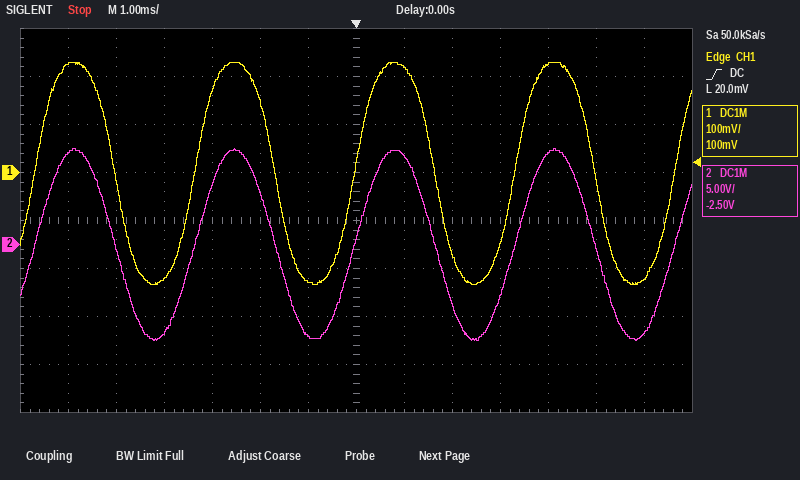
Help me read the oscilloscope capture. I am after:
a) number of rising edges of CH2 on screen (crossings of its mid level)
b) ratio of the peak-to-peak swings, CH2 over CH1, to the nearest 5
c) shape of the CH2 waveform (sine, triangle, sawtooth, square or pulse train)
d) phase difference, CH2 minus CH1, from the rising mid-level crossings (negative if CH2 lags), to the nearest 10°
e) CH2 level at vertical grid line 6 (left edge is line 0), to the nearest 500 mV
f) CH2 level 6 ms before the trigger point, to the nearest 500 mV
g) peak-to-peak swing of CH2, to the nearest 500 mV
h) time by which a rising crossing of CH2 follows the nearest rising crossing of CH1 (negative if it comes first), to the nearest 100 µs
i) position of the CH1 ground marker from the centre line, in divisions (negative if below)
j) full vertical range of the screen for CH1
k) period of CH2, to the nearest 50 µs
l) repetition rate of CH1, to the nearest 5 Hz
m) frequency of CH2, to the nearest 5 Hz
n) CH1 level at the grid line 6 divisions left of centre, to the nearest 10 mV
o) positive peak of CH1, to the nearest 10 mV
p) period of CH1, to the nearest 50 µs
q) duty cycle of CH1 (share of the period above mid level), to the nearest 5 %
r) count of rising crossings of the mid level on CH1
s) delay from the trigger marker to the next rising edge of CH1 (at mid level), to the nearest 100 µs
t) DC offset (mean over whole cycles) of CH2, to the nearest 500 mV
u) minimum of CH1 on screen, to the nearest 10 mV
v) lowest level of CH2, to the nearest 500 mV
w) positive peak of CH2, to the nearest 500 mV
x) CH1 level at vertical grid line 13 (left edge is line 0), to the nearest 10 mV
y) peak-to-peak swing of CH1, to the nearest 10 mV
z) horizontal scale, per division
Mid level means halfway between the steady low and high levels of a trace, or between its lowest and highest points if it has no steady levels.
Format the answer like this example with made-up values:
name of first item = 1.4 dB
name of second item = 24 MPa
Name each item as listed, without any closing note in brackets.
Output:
number of rising edges of CH2 on screen = 5
ratio of the peak-to-peak swings, CH2 over CH1, to the nearest 5 = 45
shape of the CH2 waveform = sine
phase difference, CH2 minus CH1, from the rising mid-level crossings (negative if CH2 lags), to the nearest 10° = 0°
CH2 level at vertical grid line 6 (left edge is line 0), to the nearest 500 mV = -9.5 V
CH2 level 6 ms before the trigger point, to the nearest 500 mV = 9.5 V
peak-to-peak swing of CH2, to the nearest 500 mV = 20.0 V
time by which a rising crossing of CH2 follows the nearest rising crossing of CH1 (negative if it comes first), to the nearest 100 µs = 0.0 ms
position of the CH1 ground marker from the centre line, in divisions = +1.0 div
full vertical range of the screen for CH1 = 800 mV
period of CH2, to the nearest 50 µs = 3.35 ms
repetition rate of CH1, to the nearest 5 Hz = 300 Hz
frequency of CH2, to the nearest 5 Hz = 300 Hz
CH1 level at the grid line 6 divisions left of centre, to the nearest 10 mV = 230 mV
positive peak of CH1, to the nearest 10 mV = 230 mV
period of CH1, to the nearest 50 µs = 3.35 ms
duty cycle of CH1 (share of the period above mid level), to the nearest 5 % = 50 %
count of rising crossings of the mid level on CH1 = 5
delay from the trigger marker to the next rising edge of CH1 (at mid level), to the nearest 100 µs = 3.3 ms
DC offset (mean over whole cycles) of CH2, to the nearest 500 mV = 0.0 V
minimum of CH1 on screen, to the nearest 10 mV = -230 mV
lowest level of CH2, to the nearest 500 mV = -10.0 V
positive peak of CH2, to the nearest 500 mV = 10.0 V
CH1 level at vertical grid line 13 (left edge is line 0), to the nearest 10 mV = -220 mV
peak-to-peak swing of CH1, to the nearest 10 mV = 460 mV
horizontal scale, per division = 1 ms
